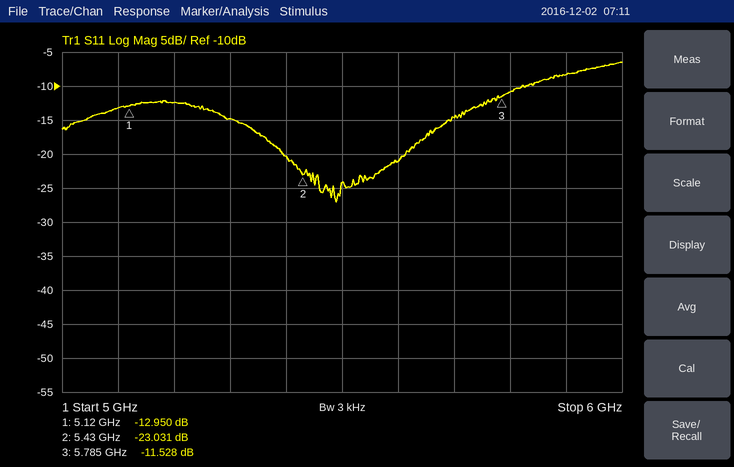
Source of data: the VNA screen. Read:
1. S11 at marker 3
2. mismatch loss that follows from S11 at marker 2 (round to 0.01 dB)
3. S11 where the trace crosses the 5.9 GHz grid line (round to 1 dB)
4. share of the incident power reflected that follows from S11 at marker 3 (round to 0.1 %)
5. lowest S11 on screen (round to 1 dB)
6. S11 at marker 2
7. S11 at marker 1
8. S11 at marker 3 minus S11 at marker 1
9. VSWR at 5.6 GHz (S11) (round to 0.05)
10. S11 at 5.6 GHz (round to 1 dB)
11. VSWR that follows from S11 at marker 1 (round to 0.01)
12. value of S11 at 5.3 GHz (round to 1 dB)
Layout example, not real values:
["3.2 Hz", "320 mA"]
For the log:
["-11.528 dB", "0.02 dB", "-8 dB", "7.0 %", "-27 dB", "-23.031 dB", "-12.950 dB", "1.422 dB", "1.20", "-21 dB", "1.58", "-15 dB"]
